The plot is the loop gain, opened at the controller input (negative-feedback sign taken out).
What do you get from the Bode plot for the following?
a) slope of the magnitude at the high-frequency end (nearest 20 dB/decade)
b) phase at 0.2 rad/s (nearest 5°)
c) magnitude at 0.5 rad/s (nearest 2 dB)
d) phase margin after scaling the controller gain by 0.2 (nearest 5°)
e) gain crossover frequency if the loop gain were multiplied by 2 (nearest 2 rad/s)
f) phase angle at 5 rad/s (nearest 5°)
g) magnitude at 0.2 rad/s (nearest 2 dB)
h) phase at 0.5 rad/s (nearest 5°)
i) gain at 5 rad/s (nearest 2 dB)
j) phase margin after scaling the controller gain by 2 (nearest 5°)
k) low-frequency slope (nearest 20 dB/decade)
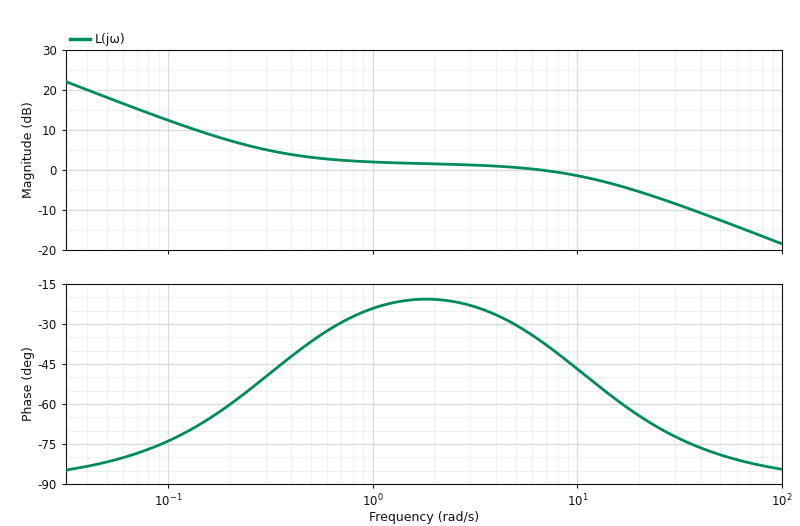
-20 dB/decade
-60°
4 dB
105°
22 rad/s
-30°
8 dB
-35°
0 dB
115°
-20 dB/decade
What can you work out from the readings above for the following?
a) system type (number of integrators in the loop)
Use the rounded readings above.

1
